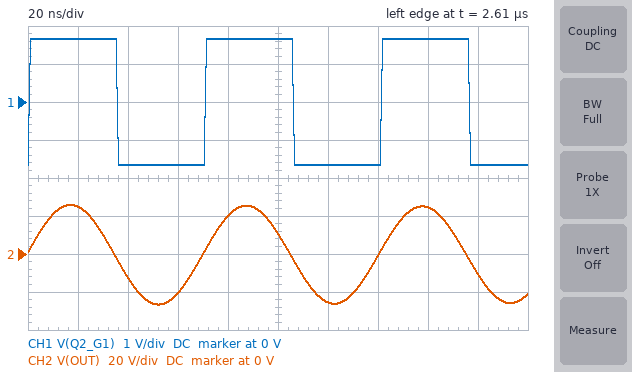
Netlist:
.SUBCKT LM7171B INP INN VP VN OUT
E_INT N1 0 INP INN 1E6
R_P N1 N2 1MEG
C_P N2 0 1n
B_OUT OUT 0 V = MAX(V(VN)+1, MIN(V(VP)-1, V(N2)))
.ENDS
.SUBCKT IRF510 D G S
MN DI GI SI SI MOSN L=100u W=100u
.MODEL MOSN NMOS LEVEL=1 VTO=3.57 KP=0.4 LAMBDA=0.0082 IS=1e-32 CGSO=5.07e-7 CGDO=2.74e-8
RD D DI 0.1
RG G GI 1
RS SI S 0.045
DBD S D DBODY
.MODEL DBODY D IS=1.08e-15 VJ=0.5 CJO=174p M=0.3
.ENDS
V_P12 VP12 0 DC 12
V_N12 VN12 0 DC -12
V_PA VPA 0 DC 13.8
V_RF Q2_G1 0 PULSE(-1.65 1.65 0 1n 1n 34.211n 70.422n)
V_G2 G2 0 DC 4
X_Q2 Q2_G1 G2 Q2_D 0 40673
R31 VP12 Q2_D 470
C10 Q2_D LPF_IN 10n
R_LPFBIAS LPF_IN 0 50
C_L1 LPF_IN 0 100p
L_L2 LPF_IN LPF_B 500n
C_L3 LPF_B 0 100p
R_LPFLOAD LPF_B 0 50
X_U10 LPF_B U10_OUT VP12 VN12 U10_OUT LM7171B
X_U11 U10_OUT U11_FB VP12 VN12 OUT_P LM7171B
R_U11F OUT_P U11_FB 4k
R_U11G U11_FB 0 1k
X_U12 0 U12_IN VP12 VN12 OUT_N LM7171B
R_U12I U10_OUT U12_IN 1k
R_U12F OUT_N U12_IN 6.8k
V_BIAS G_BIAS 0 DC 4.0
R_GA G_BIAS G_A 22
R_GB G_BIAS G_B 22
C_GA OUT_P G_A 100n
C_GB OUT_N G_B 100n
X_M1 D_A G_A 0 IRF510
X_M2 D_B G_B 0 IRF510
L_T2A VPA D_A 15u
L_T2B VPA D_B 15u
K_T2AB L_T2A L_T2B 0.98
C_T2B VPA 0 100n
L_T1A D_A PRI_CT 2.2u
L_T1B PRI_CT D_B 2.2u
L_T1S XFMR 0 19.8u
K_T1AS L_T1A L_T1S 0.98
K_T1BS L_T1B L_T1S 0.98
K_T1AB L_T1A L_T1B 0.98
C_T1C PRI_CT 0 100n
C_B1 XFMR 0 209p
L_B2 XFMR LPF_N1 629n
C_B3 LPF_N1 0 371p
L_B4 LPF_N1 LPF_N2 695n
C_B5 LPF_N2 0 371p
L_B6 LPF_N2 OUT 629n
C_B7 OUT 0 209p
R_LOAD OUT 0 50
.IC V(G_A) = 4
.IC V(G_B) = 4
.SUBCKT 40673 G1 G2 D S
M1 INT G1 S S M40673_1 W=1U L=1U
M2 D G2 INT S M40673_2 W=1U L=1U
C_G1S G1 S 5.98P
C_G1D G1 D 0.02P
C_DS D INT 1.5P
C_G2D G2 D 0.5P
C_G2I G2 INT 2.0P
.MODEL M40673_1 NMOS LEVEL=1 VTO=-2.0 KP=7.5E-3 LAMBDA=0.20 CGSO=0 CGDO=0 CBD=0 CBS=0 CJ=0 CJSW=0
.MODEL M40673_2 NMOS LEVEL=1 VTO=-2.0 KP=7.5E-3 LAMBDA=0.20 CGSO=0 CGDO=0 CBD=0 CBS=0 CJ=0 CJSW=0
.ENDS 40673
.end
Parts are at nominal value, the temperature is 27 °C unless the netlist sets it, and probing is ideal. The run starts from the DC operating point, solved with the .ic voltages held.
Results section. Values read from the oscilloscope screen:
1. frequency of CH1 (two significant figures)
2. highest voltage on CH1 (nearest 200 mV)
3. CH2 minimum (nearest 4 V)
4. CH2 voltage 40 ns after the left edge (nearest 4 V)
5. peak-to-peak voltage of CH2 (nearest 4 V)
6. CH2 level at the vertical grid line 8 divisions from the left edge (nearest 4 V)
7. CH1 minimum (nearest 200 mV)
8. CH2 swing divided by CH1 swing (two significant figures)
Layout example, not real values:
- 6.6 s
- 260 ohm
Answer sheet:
- 14 MHz
- 1.6 V
- -28 V
- -12 V
- 52 V
- 24 V
- -1.6 V
- 16
